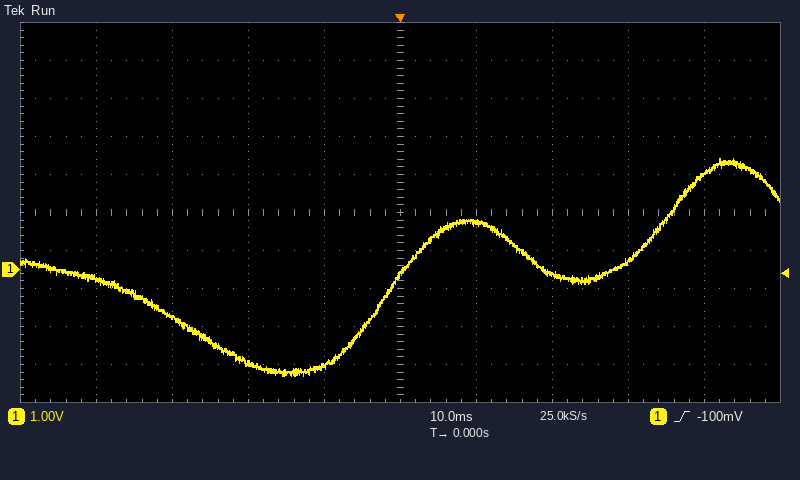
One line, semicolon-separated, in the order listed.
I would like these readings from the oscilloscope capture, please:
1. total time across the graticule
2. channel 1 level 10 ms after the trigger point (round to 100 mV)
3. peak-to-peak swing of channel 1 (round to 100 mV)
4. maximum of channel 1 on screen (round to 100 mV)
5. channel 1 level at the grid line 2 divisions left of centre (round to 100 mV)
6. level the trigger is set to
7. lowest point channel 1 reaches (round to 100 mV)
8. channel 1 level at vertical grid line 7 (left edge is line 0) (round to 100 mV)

100 ms; 1.2 V; 5.7 V; 2.9 V; -2.4 V; -100 mV; -2.8 V; -100 mV
